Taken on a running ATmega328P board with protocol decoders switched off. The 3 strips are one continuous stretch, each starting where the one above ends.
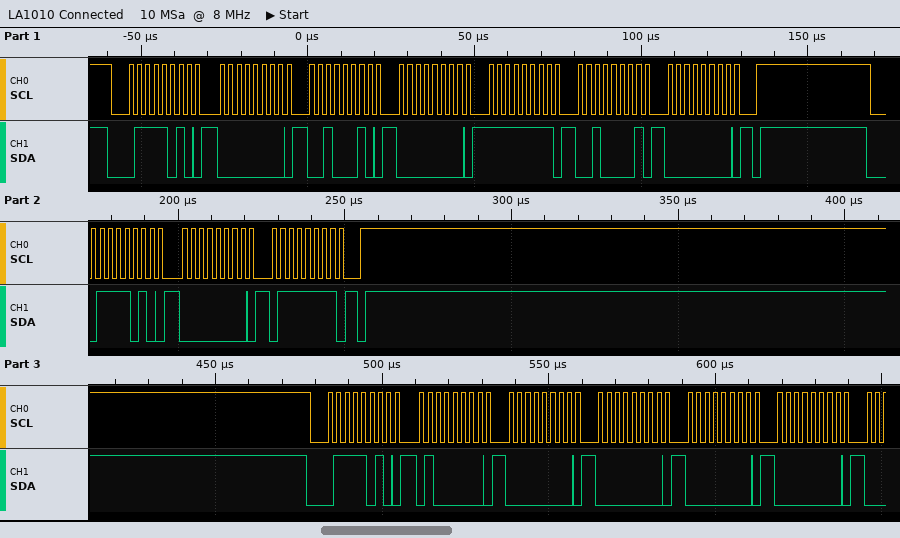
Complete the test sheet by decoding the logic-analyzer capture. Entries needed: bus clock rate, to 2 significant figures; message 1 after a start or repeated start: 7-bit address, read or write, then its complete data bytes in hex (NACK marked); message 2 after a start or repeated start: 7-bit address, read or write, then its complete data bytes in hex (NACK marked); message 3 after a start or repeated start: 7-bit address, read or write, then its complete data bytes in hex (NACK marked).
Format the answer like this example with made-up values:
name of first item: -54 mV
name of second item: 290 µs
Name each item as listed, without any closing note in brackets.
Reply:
bus clock rate, to 2 significant figures: 400 kHz
message 1 after a start or repeated start: 7-bit address, read or write, then its complete data bytes in hex: 0x3D write: 00 22 00 FF 21 00
message 2 after a start or repeated start: 7-bit address, read or write, then its complete data bytes in hex: 0x3D write: 00 7F
message 3 after a start or repeated start: 7-bit address, read or write, then its complete data bytes in hex: 0x3D write: 40 00 00 00 00
